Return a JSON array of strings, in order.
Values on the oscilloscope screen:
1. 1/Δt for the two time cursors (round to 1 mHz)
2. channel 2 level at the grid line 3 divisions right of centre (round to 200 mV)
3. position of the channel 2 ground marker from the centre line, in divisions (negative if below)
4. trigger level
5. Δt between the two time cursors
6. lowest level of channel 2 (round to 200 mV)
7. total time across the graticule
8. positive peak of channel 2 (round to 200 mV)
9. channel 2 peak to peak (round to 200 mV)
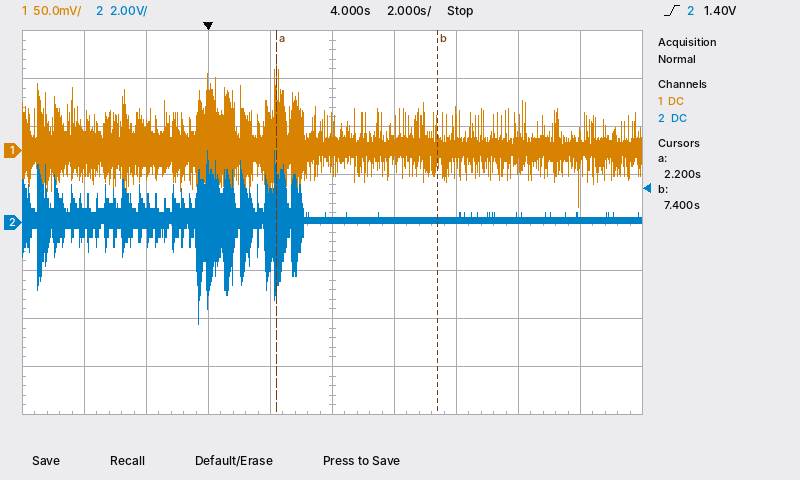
["192 mHz", "200 mV", "0.0 div", "1.40 V", "5.2 s", "-4.2 V", "20 s", "3.0 V", "7.2 V"]
